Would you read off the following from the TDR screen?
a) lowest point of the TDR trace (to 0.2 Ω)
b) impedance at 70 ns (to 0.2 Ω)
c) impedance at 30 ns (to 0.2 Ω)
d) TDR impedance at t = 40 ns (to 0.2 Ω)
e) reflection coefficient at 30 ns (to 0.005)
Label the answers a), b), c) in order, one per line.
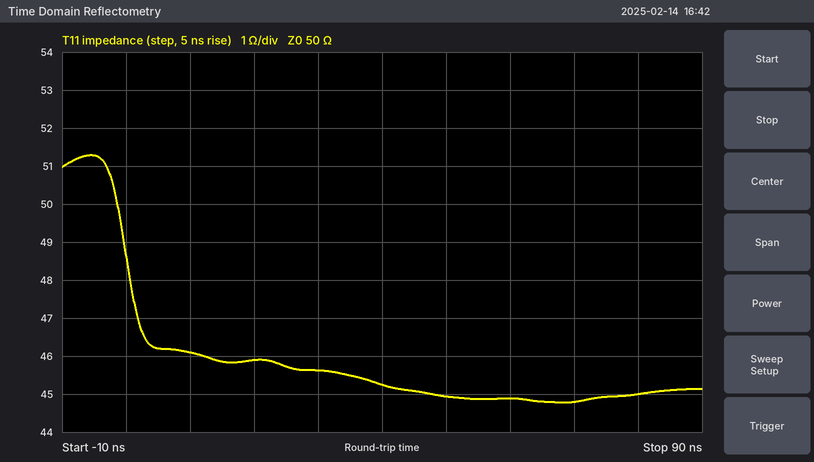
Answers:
a) 44.8 Ω
b) 44.8 Ω
c) 45.6 Ω
d) 45.2 Ω
e) -0.045
